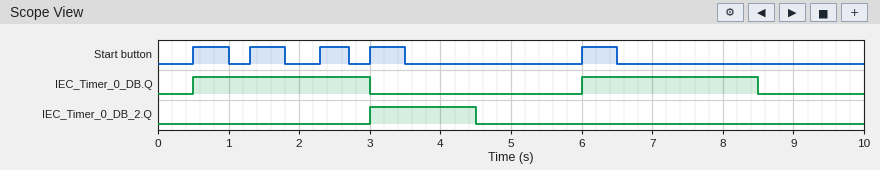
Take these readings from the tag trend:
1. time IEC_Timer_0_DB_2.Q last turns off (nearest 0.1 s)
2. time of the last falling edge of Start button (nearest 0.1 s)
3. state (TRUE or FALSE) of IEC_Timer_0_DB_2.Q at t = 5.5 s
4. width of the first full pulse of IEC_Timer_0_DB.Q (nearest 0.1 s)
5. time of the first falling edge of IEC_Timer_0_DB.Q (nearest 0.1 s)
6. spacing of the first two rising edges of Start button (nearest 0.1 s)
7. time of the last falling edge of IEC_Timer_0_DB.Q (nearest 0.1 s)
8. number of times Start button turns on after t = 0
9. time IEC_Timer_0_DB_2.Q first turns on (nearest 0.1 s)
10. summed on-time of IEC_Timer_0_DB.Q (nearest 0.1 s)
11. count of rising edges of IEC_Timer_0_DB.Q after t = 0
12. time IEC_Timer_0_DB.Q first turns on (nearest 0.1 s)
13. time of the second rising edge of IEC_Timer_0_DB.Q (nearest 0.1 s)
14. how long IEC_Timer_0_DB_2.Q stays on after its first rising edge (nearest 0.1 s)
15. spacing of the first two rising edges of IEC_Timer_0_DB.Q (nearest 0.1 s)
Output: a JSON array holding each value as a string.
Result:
["4.5 s", "6.5 s", "FALSE", "2.5 s", "3.0 s", "0.8 s", "8.5 s", "5", "3.0 s", "5.0 s", "2", "0.5 s", "6.0 s", "1.5 s", "5.5 s"]
